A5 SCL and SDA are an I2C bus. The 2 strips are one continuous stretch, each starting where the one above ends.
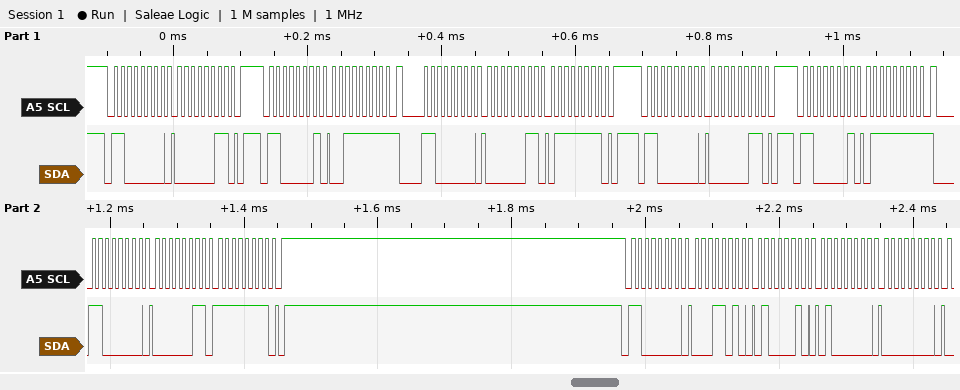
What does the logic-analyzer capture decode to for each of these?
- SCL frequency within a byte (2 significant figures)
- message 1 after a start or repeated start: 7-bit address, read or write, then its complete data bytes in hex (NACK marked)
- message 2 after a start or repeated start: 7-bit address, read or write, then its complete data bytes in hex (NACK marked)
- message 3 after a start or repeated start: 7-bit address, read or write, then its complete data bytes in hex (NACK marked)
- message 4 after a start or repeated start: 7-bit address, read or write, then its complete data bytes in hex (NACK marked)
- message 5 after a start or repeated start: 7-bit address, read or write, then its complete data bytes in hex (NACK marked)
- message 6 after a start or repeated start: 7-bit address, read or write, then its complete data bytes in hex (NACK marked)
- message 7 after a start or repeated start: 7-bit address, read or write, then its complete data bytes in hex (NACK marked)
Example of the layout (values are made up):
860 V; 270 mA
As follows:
100 kHz; 0x60 write: 03; 0x60 read: 3F NACK; 0x60 write: 03 7F; 0x60 write: 03; 0x60 read: 7F NACK; 0x60 write: 03 FF; 0x60 write: 1A 42 40 00
